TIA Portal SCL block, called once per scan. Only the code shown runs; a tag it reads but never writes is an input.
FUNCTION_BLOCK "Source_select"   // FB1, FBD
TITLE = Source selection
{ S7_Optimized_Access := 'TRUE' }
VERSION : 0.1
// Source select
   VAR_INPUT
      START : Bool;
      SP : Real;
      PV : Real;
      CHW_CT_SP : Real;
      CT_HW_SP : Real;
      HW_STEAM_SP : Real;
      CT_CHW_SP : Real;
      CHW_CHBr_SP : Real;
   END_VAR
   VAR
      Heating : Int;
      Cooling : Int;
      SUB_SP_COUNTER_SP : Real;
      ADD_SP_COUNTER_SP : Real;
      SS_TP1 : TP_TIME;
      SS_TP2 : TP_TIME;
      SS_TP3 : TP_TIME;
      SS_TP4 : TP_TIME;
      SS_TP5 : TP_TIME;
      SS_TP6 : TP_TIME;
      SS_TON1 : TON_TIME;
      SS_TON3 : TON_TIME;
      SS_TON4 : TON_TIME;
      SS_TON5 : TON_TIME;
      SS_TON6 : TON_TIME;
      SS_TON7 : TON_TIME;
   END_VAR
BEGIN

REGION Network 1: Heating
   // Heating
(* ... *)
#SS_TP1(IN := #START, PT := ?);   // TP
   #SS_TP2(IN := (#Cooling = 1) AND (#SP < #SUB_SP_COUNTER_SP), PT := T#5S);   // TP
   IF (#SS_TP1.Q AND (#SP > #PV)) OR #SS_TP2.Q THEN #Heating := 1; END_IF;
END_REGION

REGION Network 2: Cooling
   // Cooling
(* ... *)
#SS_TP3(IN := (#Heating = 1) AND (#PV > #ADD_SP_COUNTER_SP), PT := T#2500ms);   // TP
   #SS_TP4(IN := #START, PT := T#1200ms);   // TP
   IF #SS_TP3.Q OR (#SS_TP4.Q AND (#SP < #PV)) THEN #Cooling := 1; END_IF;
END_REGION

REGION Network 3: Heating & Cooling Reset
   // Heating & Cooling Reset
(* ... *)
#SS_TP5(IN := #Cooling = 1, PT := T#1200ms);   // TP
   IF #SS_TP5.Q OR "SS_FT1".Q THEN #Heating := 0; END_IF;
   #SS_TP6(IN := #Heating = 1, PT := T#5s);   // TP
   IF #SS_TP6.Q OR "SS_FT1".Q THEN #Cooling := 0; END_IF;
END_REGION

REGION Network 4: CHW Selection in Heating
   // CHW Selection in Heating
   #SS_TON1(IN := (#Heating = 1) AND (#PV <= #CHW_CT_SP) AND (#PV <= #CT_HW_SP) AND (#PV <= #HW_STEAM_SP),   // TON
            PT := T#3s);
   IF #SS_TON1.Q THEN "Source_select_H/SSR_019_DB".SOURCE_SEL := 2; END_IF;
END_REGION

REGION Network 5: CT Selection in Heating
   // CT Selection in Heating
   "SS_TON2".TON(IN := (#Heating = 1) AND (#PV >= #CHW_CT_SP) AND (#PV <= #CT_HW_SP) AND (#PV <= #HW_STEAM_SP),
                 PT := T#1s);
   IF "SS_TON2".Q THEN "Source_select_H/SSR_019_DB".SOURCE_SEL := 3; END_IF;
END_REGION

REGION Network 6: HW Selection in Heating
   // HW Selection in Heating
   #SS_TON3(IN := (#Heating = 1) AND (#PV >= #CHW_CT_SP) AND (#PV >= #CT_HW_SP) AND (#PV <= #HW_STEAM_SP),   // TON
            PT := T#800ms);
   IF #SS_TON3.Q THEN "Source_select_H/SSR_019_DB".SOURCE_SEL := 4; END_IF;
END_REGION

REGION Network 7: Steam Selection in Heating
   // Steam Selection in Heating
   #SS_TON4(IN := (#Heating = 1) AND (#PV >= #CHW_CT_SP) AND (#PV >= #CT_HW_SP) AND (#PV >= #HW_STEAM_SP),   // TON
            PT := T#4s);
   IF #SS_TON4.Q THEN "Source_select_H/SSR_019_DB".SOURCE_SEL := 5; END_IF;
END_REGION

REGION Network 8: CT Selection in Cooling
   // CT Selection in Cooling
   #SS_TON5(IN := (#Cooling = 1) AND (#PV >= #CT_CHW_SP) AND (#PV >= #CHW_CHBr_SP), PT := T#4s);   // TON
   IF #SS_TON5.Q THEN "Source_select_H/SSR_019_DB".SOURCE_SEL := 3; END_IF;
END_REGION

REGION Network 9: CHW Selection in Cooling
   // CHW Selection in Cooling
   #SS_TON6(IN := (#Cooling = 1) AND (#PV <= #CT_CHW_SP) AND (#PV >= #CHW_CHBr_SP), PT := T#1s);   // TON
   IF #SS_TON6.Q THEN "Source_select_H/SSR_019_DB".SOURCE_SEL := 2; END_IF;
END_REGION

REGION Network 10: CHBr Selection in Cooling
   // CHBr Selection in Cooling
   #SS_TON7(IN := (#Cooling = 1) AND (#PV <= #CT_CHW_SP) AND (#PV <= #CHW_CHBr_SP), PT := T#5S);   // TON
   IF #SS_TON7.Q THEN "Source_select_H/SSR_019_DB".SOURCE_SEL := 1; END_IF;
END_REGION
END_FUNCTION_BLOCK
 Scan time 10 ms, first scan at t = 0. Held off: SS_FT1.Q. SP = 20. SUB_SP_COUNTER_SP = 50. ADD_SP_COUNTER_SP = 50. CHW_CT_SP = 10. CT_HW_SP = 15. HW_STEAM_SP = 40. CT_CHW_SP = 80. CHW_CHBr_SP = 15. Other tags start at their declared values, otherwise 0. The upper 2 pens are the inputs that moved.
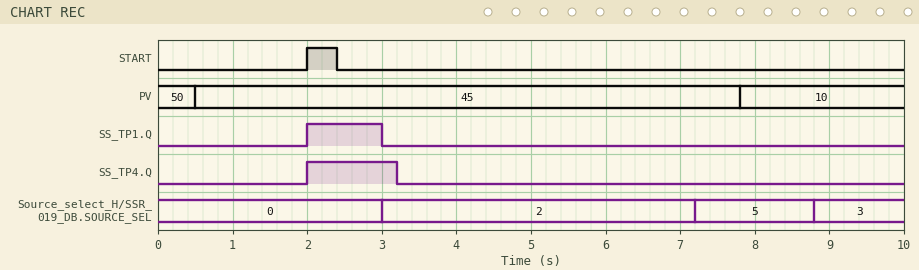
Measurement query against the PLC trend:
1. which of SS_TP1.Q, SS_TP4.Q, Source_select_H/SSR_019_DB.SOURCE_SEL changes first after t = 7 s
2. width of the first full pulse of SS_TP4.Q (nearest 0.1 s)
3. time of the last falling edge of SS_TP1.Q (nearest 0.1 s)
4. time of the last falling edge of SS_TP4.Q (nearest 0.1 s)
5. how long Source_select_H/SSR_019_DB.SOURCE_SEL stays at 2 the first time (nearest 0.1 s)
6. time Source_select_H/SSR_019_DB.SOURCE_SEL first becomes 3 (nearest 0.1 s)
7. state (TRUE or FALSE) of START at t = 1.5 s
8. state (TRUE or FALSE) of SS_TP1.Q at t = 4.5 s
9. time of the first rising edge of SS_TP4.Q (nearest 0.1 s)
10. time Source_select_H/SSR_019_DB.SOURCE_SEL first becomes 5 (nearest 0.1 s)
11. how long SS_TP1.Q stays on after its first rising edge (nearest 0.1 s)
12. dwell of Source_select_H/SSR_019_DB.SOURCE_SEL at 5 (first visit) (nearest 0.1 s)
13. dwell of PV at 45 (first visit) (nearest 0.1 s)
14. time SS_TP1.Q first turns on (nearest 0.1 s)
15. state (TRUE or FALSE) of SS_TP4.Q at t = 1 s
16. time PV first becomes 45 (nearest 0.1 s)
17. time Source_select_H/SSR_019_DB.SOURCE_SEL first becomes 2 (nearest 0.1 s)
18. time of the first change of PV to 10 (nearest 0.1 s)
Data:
Source_select_H/SSR_019_DB.SOURCE_SEL
1.2 s
3.0 s
3.2 s
4.2 s
8.8 s
FALSE
FALSE
2.0 s
7.2 s
1.0 s
1.6 s
7.3 s
2.0 s
FALSE
0.5 s
3.0 s
7.8 s
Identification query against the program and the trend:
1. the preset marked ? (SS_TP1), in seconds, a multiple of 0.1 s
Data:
1.0 s
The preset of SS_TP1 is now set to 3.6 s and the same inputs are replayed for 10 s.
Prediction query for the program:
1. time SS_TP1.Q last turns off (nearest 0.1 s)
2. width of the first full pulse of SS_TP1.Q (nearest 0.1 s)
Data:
5.6 s
3.6 s
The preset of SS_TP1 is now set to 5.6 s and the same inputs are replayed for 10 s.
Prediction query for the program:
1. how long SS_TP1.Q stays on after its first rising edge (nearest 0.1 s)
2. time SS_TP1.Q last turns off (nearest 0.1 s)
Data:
5.6 s
7.6 s
